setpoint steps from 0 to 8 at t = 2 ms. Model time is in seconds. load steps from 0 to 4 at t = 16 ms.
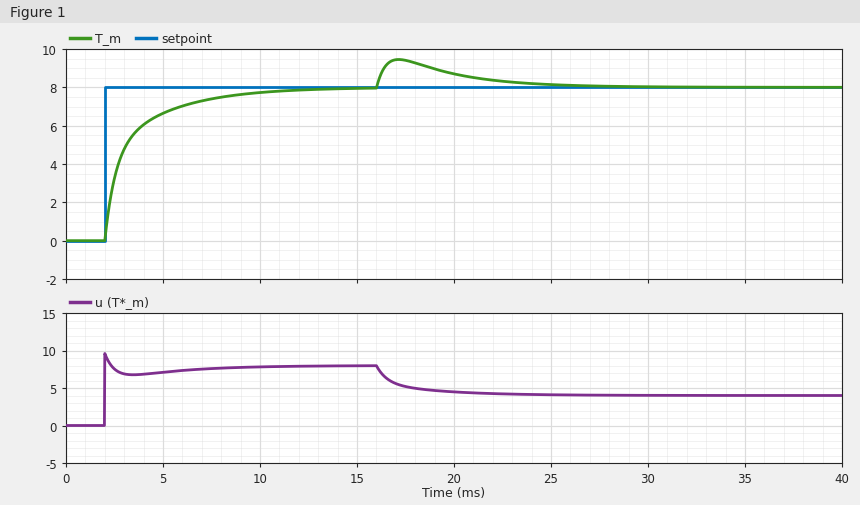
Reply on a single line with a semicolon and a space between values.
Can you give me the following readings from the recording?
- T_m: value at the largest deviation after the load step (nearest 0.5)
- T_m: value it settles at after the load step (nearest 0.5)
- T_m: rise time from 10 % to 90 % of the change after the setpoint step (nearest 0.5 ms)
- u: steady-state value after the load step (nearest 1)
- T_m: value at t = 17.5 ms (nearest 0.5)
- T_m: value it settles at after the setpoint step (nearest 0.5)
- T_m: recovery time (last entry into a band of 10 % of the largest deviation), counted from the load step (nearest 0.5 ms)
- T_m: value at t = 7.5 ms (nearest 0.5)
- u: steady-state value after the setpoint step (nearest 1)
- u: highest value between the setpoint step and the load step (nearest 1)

9.5; 8.0; 4.5 ms; 4; 9.5; 8.0; 9.0 ms; 7.5; 8; 10
